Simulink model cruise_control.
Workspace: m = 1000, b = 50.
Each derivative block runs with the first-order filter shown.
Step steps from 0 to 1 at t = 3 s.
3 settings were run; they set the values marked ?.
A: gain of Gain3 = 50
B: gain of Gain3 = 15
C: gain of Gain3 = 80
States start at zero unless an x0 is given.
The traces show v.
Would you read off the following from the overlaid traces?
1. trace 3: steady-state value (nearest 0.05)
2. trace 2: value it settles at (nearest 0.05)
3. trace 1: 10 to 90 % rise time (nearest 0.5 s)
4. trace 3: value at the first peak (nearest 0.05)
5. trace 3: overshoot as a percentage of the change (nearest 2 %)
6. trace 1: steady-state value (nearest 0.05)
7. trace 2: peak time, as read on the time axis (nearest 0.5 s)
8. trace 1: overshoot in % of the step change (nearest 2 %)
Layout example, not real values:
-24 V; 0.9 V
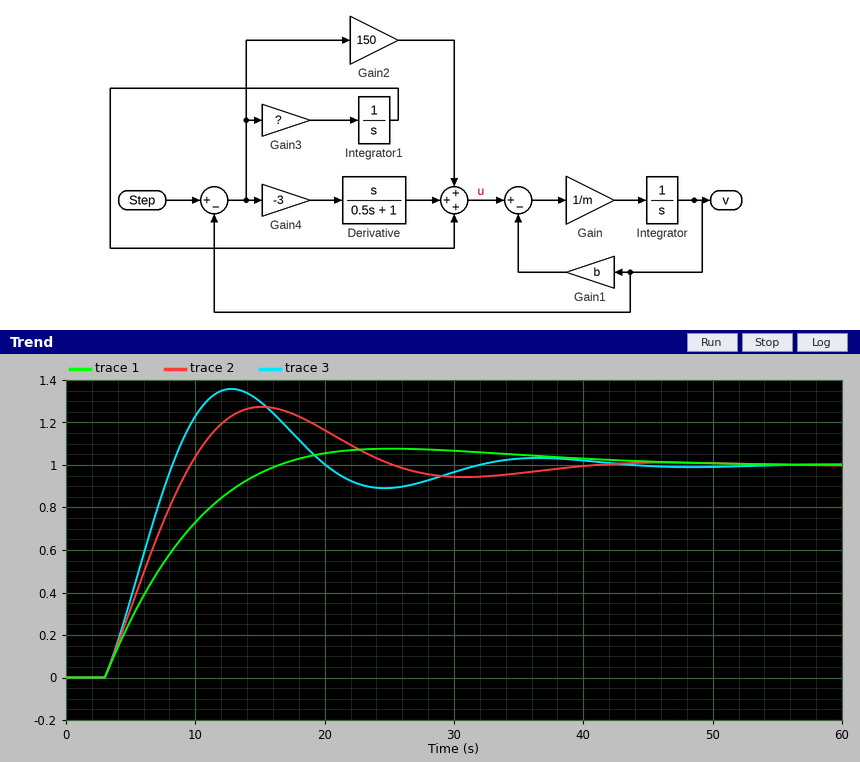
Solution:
1.00; 1.00; 9.5 s; 1.35; 36 %; 1.00; 15.0 s; 8 %
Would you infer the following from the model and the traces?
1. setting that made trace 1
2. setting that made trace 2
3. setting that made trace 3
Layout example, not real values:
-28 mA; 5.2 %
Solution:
B; A; C
